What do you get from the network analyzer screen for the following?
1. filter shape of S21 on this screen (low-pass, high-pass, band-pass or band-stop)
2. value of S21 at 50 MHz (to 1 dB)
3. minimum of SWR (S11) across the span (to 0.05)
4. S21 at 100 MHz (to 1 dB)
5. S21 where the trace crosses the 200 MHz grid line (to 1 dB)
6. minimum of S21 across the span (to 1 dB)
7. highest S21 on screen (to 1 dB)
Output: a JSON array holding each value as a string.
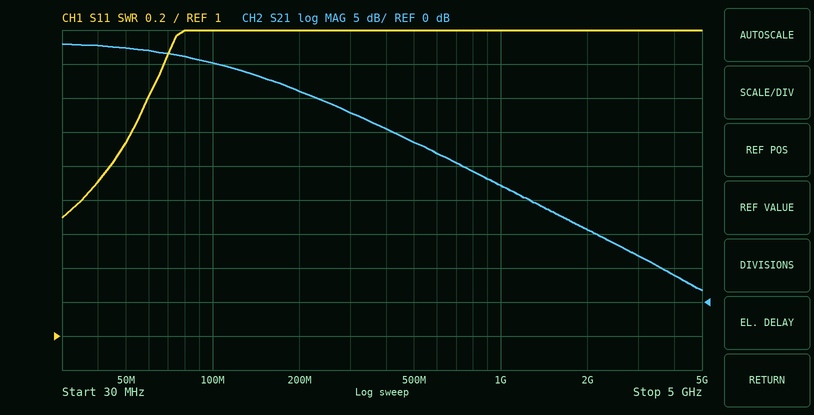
["low-pass", "37 dB", "1.70", "35 dB", "31 dB", "2 dB", "38 dB"]
